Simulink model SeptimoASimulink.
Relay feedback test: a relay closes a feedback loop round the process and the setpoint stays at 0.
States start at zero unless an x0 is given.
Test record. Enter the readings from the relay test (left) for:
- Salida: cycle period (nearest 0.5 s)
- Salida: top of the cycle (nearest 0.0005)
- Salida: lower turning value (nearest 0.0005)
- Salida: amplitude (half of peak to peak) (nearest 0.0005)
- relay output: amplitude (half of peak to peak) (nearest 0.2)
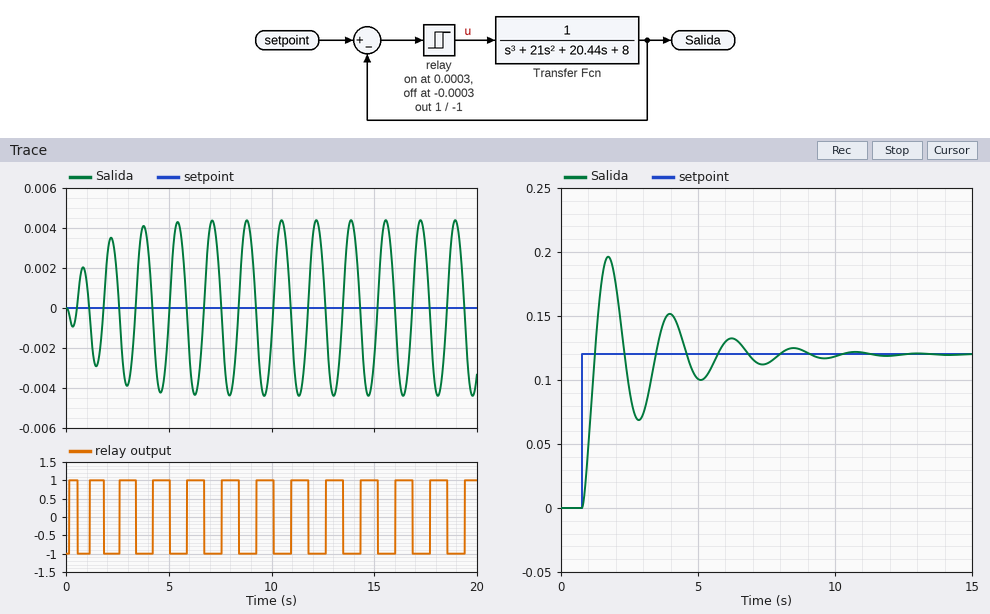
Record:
1.5 s
0.0045
-0.0045
0.0045
1.0
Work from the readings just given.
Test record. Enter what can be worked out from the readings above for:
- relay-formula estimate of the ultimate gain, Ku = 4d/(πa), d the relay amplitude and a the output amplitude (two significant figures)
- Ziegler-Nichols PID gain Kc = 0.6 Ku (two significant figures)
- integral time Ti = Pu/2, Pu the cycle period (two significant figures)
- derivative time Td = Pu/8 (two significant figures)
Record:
280
170
0.75 s
0.19 s
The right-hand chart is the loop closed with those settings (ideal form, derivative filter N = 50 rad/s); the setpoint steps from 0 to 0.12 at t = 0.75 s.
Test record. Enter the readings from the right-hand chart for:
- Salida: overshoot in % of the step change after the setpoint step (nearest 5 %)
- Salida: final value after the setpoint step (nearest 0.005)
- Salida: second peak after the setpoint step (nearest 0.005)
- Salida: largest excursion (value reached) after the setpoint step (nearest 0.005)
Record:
65 %
0.120
0.150
0.195
